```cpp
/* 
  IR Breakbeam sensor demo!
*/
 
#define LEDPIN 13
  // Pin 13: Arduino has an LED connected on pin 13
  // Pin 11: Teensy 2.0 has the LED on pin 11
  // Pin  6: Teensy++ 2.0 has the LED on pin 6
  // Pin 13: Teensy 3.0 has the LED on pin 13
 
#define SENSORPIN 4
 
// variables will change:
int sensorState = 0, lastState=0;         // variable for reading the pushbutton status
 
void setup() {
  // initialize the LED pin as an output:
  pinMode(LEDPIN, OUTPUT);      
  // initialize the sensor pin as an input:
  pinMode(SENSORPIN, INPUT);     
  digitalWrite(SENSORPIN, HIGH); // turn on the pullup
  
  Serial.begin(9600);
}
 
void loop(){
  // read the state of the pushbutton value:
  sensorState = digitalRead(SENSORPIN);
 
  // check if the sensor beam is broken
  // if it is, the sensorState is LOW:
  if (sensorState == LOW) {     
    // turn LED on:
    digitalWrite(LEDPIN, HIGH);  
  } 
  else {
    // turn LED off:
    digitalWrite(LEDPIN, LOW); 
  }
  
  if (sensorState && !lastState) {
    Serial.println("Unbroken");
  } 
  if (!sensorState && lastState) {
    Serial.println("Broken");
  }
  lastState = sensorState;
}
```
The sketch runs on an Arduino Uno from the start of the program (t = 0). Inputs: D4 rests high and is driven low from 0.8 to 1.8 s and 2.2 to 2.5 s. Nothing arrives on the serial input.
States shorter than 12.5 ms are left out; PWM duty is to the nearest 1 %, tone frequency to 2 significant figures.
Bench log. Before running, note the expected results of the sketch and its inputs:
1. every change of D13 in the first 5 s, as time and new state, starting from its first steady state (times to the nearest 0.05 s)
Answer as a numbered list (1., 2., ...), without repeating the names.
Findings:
1. 0 s low; 0.8 s high; 1.8 s low; 2.2 s high; 2.5 s low
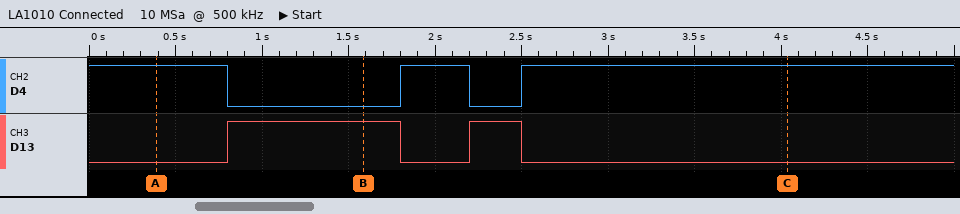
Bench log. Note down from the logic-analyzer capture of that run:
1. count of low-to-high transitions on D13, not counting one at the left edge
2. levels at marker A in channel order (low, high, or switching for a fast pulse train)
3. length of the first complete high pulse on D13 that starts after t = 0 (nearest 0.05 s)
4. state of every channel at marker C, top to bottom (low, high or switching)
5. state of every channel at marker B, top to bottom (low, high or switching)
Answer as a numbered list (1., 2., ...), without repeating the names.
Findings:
1. 2
2. D4 high, D13 low
3. 1.00 s
4. D4 high, D13 low
5. D4 low, D13 high
